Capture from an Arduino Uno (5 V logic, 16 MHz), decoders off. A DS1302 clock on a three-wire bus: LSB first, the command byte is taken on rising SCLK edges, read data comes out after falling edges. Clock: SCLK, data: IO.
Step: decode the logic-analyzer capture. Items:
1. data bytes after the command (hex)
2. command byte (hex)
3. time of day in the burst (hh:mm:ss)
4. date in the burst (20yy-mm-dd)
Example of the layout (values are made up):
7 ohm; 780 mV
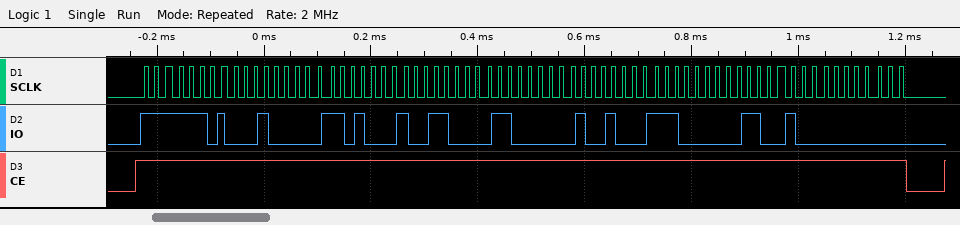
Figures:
08 16 19 06 12 07 26 00; 0xBF; 19:16:08; 2026-12-06
